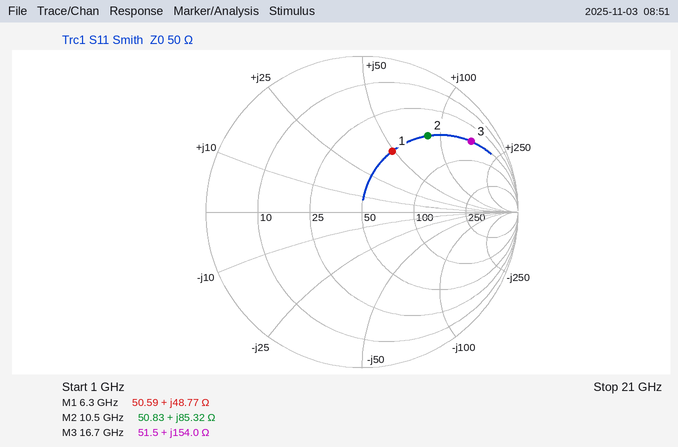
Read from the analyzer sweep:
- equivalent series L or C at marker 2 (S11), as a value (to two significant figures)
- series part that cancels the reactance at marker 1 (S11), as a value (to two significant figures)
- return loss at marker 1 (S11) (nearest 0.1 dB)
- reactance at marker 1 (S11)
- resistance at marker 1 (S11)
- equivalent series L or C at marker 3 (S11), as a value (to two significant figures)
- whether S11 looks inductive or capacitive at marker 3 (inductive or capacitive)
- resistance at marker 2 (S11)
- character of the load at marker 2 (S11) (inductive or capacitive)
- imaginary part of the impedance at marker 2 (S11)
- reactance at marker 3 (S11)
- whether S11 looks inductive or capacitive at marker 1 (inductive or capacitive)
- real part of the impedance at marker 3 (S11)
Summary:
1.3 nH
520 fF
7.2 dB
+48.77 Ω
50.59 Ω
1.5 nH
inductive
50.83 Ω
inductive
+85.32 Ω
+154.0 Ω
inductive
51.5 Ω
